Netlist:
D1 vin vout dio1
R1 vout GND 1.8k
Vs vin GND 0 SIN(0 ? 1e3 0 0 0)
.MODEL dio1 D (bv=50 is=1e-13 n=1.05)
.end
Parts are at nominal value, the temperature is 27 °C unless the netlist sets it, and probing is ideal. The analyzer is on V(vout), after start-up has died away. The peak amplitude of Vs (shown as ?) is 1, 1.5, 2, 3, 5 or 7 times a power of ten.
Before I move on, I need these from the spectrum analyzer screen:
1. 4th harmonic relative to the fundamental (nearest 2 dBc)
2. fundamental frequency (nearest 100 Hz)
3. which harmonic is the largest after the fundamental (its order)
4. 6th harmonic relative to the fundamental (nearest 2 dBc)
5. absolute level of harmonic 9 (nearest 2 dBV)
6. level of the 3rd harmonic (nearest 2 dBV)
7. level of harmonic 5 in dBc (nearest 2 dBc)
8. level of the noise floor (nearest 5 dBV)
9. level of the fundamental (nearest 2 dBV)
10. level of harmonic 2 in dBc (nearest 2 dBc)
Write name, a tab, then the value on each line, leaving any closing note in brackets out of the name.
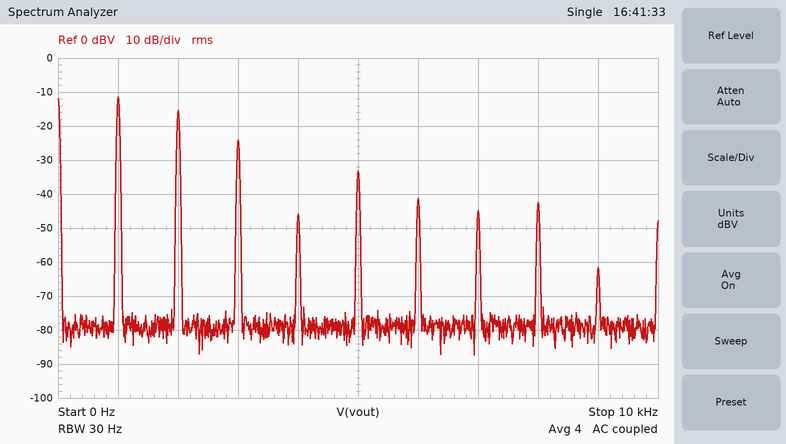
4th harmonic relative to the fundamental	-34 dBc
fundamental frequency	1.0 kHz
which harmonic is the largest after the fundamental	2
6th harmonic relative to the fundamental	-30 dBc
absolute level of harmonic 9	-62 dBV
level of the 3rd harmonic	-24 dBV
level of harmonic 5 in dBc	-22 dBc
level of the noise floor	-80 dBV
level of the fundamental	-12 dBV
level of harmonic 2 in dBc	-4 dBc
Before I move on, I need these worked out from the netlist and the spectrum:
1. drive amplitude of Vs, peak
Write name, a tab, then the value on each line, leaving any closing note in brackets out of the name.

drive amplitude of Vs, peak	1.5 V
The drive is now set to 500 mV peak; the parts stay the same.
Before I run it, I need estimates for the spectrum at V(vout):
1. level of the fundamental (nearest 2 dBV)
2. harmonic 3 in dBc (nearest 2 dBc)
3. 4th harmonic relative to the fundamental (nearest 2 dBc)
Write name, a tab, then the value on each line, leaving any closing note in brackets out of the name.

level of the fundamental	-56 dBV
harmonic 3 in dBc	-2 dBc
4th harmonic relative to the fundamental	-4 dBc
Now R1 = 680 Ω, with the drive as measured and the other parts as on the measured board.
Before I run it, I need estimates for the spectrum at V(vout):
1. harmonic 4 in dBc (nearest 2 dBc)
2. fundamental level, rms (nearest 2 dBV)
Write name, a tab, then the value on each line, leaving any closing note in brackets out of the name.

harmonic 4 in dBc	-40 dBc
fundamental level, rms	-12 dBV
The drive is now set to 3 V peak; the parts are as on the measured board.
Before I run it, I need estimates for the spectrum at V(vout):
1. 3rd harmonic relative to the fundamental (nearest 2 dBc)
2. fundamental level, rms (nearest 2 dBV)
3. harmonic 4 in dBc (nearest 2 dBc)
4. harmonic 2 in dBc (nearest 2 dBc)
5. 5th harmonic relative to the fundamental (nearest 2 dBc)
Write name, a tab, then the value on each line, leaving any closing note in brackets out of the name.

3rd harmonic relative to the fundamental	-20 dBc
fundamental level, rms	-2 dBV
harmonic 4 in dBc	-22 dBc
harmonic 2 in dBc	-6 dBc
5th harmonic relative to the fundamental	-26 dBc
